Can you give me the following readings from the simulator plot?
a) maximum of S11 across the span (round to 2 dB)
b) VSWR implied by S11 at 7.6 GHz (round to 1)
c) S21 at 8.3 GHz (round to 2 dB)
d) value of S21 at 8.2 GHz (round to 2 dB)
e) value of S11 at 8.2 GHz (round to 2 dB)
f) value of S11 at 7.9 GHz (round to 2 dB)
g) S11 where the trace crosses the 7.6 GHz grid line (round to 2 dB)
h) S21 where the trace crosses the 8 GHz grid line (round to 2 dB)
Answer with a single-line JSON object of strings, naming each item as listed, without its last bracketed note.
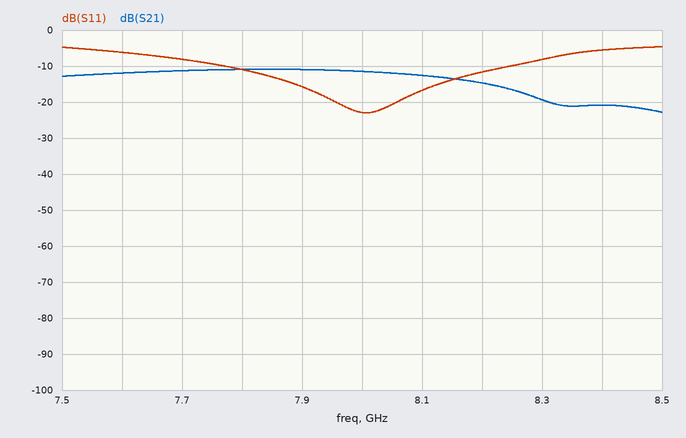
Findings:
{"maximum of S11 across the span": "-4 dB", "VSWR implied by S11 at 7.6 GHz": "3", "S21 at 8.3 GHz": "-20 dB", "value of S21 at 8.2 GHz": "-14 dB", "value of S11 at 8.2 GHz": "-12 dB", "value of S11 at 7.9 GHz": "-16 dB", "S11 where the trace crosses the 7.6 GHz grid line": "-6 dB", "S21 where the trace crosses the 8 GHz grid line": "-12 dB"}
